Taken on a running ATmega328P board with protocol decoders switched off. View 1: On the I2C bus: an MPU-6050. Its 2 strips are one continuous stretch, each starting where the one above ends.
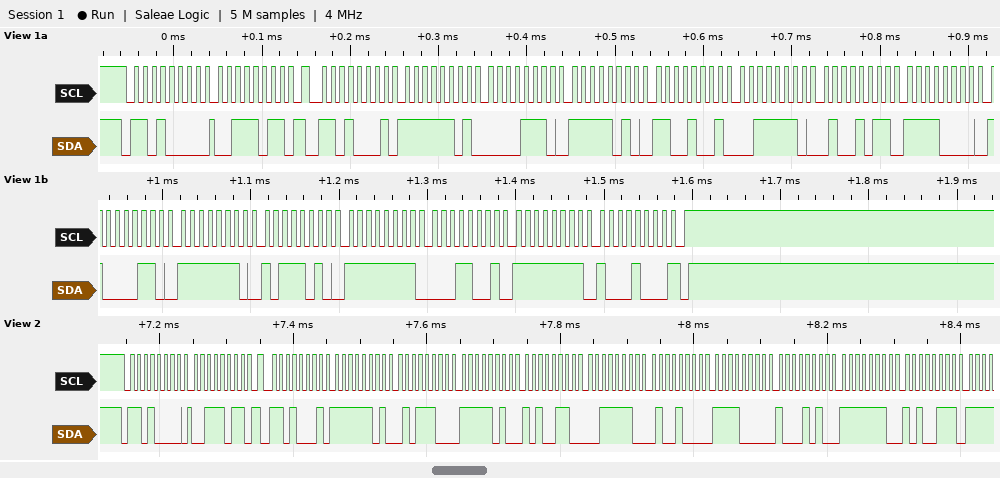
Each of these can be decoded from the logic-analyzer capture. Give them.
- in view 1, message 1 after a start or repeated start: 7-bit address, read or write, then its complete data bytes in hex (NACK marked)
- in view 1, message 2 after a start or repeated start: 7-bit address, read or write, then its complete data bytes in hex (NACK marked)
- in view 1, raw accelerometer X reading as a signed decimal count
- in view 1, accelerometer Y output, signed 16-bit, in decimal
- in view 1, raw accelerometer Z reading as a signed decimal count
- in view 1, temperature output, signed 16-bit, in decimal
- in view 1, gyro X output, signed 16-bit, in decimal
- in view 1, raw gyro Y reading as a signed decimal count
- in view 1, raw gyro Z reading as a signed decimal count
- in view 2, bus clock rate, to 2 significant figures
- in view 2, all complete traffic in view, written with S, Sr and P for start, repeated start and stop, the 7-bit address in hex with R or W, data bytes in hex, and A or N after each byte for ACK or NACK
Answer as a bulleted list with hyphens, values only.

- 0x68 write: 3B
- 0x68 read: FD 0E FA C9 3E 4B F0 86 FE BA FF 19 FF 88 NACK
- -754
- -1335
- 15947
- -3962
- -326
- -231
- -120
- 100 kHz
- S 68W A 3B A Sr 68R A FD A 5C A FA A A6 A 3E A 48 A F0 A 8A A FE A A7 A
